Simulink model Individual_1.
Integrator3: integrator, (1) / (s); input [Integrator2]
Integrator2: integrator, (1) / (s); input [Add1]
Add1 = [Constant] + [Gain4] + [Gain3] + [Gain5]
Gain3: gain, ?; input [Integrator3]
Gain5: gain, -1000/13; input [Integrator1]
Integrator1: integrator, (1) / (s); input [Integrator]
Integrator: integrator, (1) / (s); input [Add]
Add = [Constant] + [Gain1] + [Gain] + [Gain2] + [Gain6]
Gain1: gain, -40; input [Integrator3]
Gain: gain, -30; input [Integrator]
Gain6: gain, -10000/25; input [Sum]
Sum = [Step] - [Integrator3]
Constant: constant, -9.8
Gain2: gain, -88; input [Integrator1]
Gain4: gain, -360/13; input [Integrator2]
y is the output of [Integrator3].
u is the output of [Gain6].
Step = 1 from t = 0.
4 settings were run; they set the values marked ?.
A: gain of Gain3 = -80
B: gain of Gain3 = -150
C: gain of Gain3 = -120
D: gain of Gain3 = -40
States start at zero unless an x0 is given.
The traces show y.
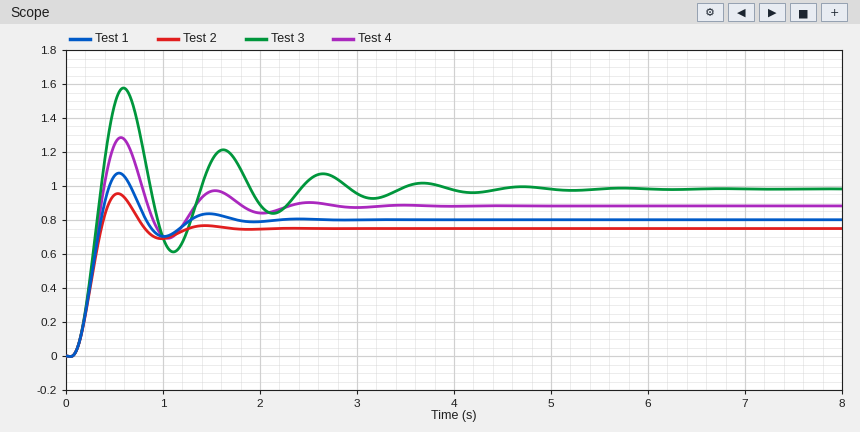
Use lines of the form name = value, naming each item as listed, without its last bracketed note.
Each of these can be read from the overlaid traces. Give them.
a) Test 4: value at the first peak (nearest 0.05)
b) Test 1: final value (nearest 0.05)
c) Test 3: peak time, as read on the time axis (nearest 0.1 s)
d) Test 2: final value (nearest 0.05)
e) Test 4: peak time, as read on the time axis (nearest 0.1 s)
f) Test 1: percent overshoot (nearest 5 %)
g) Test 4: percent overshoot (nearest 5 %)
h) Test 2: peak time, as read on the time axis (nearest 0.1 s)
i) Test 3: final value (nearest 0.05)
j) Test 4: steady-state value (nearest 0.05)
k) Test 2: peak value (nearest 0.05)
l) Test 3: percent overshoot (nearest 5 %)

Test 4: value at the first peak = 1.30
Test 1: final value = 0.80
Test 3: peak time, as read on the time axis = 0.6 s
Test 2: final value = 0.75
Test 4: peak time, as read on the time axis = 0.6 s
Test 1: percent overshoot = 35 %
Test 4: percent overshoot = 45 %
Test 2: peak time, as read on the time axis = 0.5 s
Test 3: final value = 1.00
Test 4: steady-state value = 0.90
Test 2: peak value = 0.95
Test 3: percent overshoot = 60 %
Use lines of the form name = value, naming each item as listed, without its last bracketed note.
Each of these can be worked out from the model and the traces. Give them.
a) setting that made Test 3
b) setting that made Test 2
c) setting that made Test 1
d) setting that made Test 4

setting that made Test 3 = D
setting that made Test 2 = B
setting that made Test 1 = C
setting that made Test 4 = A
